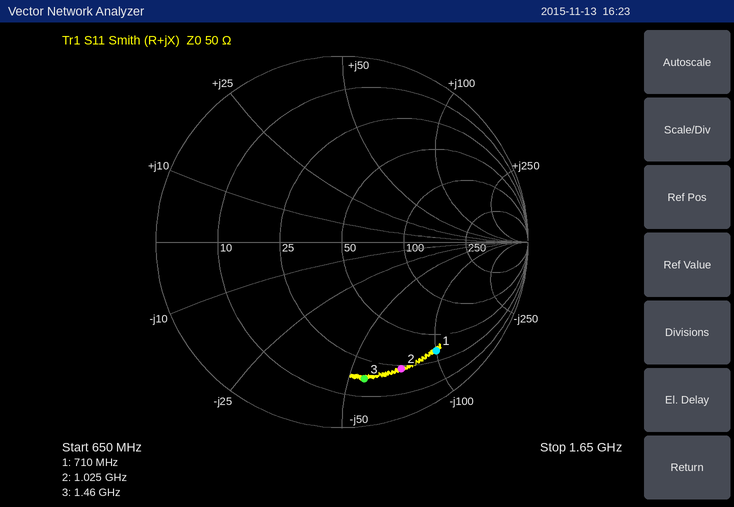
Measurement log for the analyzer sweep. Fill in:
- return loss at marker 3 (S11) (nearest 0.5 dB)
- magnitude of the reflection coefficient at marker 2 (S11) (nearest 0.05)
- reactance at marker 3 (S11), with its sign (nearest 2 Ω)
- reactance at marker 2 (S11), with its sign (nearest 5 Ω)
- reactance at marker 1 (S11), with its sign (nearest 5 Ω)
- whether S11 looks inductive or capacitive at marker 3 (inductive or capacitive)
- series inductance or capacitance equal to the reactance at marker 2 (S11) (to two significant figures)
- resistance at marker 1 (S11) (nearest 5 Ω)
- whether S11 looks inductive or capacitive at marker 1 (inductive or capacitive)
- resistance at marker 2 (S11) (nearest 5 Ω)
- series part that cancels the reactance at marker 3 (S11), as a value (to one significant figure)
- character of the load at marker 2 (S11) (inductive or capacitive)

2.5 dB
0.75
-56 Ω
-75 Ω
-100 Ω
capacitive
2.1 pF
35 Ω
capacitive
25 Ω
6 nH
capacitive
